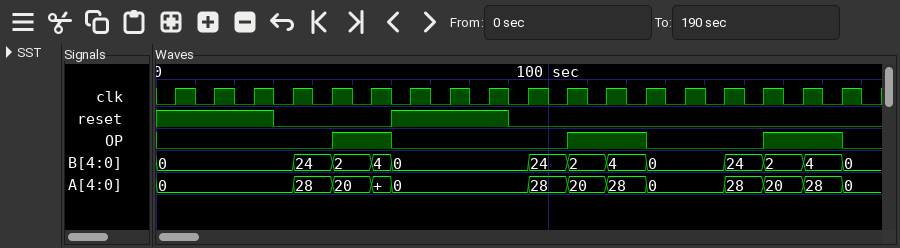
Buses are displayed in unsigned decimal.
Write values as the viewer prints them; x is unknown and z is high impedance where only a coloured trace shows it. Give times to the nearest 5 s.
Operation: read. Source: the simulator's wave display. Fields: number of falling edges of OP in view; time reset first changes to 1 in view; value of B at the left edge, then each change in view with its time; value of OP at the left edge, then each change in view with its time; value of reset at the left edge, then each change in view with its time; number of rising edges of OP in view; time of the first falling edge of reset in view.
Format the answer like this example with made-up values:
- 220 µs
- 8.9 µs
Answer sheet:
- 3
- 60 s
- 0, 24 at 35 s, 2 at 45 s, 4 at 55 s, 0 at 60 s, 24 at 95 s, 2 at 105 s, 4 at 115 s, 0 at 125 s, 24 at 145 s, 2 at 155 s, 4 at 165 s, 0 at 175 s
- 0, 1 at 45 s, 0 at 60 s, 1 at 105 s, 0 at 125 s, 1 at 155 s, 0 at 175 s
- 1, 0 at 30 s, 1 at 60 s, 0 at 90 s
- 3
- 30 s
